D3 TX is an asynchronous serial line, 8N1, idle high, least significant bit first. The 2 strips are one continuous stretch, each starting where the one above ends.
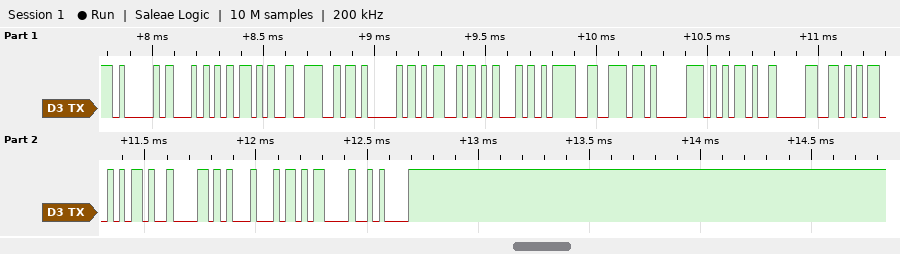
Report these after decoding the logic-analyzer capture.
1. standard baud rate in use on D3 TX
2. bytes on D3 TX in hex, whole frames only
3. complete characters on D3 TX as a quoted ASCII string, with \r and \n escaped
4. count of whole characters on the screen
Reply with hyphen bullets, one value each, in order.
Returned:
- 38400 baud
- 41 54 2B 4E 41 4D 45 3D 6E 70 2D 30 35 2D 58 44 0D 0A
- "AT+NAME=np-05-XD\r\n"
- 18
